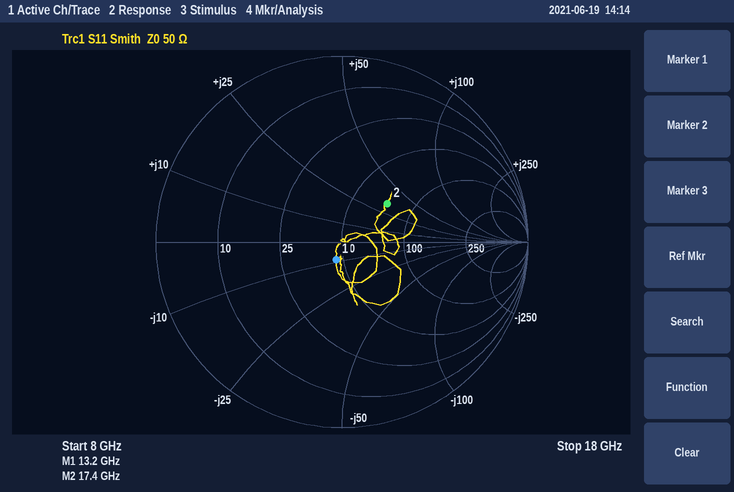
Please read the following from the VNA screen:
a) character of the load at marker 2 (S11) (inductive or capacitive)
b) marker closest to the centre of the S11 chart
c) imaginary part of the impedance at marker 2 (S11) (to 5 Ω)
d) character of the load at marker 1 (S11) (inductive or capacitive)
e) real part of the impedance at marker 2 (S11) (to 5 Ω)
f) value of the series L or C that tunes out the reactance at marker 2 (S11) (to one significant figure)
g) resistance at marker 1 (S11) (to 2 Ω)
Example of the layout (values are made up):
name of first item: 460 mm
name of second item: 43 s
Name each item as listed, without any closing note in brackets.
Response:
character of the load at marker 2 (S11): inductive
marker closest to the centre of the S11 chart: marker 1
imaginary part of the impedance at marker 2 (S11): +35 Ω
character of the load at marker 1 (S11): capacitive
real part of the impedance at marker 2 (S11): 75 Ω
value of the series L or C that tunes out the reactance at marker 2 (S11): 300 fF
resistance at marker 1 (S11): 46 Ω
